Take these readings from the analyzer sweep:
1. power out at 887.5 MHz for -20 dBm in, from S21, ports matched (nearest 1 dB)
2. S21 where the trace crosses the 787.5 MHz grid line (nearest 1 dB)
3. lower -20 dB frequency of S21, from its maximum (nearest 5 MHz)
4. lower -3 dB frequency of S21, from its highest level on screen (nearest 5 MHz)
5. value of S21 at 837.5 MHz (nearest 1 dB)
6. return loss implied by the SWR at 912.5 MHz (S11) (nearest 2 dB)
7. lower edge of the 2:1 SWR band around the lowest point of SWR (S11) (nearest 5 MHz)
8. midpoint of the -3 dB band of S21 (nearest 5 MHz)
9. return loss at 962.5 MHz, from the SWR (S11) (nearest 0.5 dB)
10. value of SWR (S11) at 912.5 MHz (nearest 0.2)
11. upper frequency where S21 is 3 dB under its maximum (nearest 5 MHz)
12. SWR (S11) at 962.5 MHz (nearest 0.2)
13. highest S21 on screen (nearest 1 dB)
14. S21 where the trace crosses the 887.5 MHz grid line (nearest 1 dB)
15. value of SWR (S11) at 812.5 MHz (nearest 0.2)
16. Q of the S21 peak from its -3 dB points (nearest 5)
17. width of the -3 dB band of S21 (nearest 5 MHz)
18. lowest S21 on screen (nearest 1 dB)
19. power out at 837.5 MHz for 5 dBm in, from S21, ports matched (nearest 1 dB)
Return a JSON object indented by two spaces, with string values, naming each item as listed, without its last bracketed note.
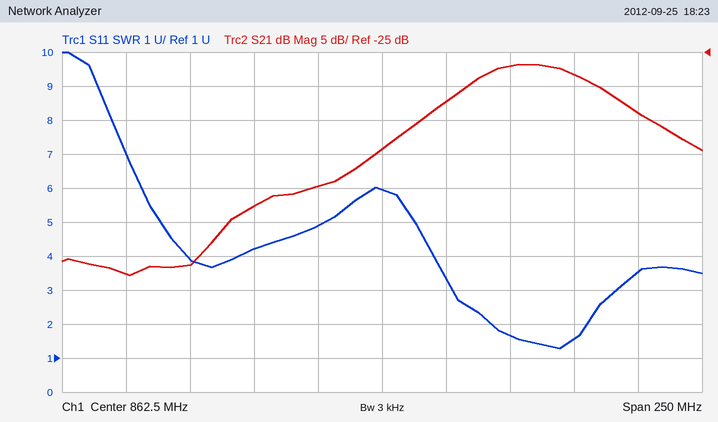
{
  "power out at 887.5 MHz for -20 dBm in, from S21, ports matched": "-52 dBm",
  "S21 where the trace crosses the 787.5 MHz grid line": "-56 dB",
  "lower -20 dB frequency of S21, from its maximum": "815 MHz",
  "lower -3 dB frequency of S21, from its highest level on screen": "895 MHz",
  "value of S21 at 837.5 MHz": "-45 dB",
  "return loss implied by the SWR at 912.5 MHz (S11)": "12 dB",
  "lower edge of the 2:1 SWR band around the lowest point of SWR (S11)": "905 MHz",
  "midpoint of the -3 dB band of S21": "920 MHz",
  "return loss at 962.5 MHz, from the SWR (S11)": "5.0 dB",
  "value of SWR (S11) at 912.5 MHz": "1.6",
  "upper frequency where S21 is 3 dB under its maximum": "945 MHz",
  "SWR (S11) at 962.5 MHz": "3.6",
  "highest S21 on screen": "-27 dB",
  "S21 where the trace crosses the 887.5 MHz grid line": "-32 dB",
  "value of SWR (S11) at 812.5 MHz": "4.2",
  "Q of the S21 peak from its -3 dB points": "20",
  "width of the -3 dB band of S21": "50 MHz",
  "lowest S21 on screen": "-58 dB",
  "power out at 837.5 MHz for 5 dBm in, from S21, ports matched": "-40 dBm"
}
